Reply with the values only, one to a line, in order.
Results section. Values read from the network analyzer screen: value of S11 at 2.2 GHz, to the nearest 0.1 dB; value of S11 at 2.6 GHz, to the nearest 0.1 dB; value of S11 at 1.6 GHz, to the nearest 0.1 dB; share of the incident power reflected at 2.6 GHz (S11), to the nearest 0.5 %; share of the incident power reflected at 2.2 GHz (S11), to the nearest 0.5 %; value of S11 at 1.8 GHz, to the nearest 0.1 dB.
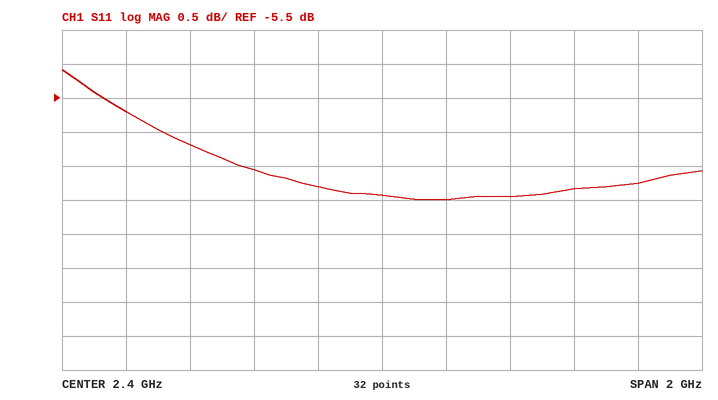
-6.8 dB
-7.0 dB
-5.7 dB
20.0 %
21.0 %
-6.2 dB
